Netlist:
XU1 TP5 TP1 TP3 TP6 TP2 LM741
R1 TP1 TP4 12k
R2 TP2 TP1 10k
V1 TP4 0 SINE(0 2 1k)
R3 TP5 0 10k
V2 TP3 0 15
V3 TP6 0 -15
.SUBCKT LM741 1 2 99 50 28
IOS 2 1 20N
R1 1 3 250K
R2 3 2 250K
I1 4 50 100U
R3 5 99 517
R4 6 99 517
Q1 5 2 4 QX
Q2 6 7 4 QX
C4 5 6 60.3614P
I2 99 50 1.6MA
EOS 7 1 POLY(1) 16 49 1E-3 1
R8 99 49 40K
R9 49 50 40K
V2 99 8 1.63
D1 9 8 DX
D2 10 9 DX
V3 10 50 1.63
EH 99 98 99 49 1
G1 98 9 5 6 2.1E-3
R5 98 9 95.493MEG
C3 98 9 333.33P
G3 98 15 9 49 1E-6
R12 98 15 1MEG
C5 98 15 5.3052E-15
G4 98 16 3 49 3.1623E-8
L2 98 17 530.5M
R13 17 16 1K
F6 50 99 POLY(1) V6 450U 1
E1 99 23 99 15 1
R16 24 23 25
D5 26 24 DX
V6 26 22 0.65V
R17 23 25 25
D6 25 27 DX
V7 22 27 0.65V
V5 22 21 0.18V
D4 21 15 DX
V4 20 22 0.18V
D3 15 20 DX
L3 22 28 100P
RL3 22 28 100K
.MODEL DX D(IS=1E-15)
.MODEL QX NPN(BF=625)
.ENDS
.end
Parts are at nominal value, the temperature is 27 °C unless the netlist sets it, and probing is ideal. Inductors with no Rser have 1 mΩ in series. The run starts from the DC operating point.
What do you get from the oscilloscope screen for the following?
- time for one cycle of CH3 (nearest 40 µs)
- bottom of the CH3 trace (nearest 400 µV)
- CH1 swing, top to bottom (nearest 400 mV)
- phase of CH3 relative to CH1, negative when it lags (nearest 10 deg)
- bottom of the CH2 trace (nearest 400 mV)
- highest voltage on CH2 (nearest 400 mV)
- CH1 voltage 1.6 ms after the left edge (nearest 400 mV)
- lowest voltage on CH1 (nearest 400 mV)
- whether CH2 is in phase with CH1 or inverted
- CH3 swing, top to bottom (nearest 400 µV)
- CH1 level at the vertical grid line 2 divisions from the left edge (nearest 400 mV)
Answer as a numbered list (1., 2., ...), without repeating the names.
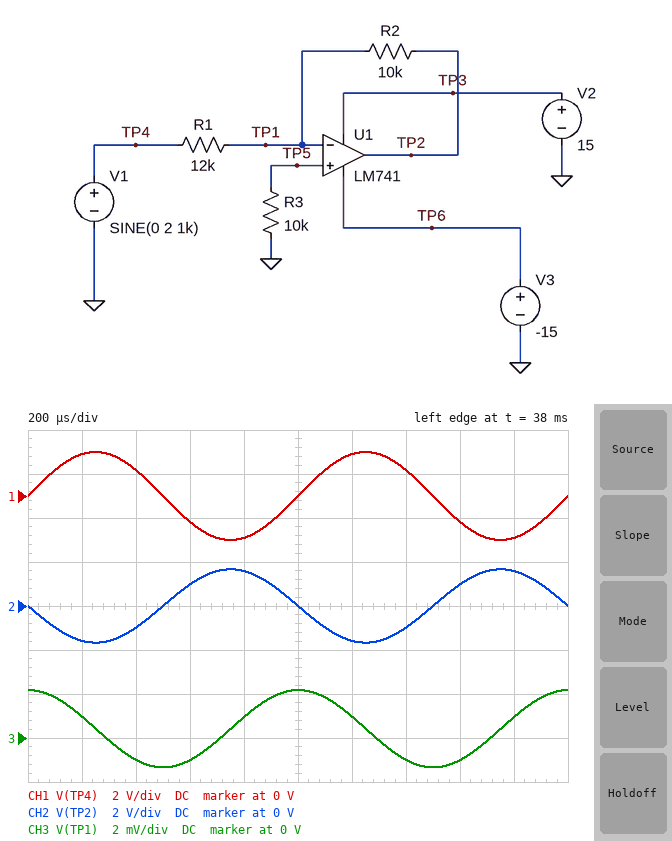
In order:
1. 1.00 ms
2. -1.2 mV
3. 4.0 V
4. 90 deg
5. -1.6 V
6. 1.6 V
7. -1.2 V
8. -2.0 V
9. inverted
10. 3.6 mV
11. 1.2 V
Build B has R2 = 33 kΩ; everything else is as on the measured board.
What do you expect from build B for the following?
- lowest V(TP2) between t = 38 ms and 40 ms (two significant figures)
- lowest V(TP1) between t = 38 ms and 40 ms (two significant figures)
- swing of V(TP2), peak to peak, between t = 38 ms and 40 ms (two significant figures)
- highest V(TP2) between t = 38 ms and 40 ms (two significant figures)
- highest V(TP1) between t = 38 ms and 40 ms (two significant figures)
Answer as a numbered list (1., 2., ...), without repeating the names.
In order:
1. -5.5 V
2. -5.3 mV
3. 11 V
4. 5.5 V
5. 6.2 mV
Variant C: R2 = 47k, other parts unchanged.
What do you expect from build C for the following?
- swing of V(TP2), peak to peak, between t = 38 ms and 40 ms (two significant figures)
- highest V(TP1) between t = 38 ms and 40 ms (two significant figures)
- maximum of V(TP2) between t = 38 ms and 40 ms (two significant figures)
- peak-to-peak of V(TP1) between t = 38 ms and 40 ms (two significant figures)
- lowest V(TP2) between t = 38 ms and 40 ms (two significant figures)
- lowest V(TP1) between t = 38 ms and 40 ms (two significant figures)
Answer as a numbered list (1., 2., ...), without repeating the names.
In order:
1. 16 V
2. 8.6 mV
3. 7.8 V
4. 16 mV
5. -7.8 V
6. -7.8 mV
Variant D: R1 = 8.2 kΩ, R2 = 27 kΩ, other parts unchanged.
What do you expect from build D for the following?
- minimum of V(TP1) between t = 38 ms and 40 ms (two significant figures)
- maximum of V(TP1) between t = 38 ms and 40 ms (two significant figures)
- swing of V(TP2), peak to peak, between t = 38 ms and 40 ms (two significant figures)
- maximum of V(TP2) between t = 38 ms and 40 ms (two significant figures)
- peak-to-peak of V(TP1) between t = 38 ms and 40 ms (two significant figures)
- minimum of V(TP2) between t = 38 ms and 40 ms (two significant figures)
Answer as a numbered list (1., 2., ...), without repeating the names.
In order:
1. -6.5 mV
2. 7.3 mV
3. 13 V
4. 6.6 V
5. 14 mV
6. -6.6 V
